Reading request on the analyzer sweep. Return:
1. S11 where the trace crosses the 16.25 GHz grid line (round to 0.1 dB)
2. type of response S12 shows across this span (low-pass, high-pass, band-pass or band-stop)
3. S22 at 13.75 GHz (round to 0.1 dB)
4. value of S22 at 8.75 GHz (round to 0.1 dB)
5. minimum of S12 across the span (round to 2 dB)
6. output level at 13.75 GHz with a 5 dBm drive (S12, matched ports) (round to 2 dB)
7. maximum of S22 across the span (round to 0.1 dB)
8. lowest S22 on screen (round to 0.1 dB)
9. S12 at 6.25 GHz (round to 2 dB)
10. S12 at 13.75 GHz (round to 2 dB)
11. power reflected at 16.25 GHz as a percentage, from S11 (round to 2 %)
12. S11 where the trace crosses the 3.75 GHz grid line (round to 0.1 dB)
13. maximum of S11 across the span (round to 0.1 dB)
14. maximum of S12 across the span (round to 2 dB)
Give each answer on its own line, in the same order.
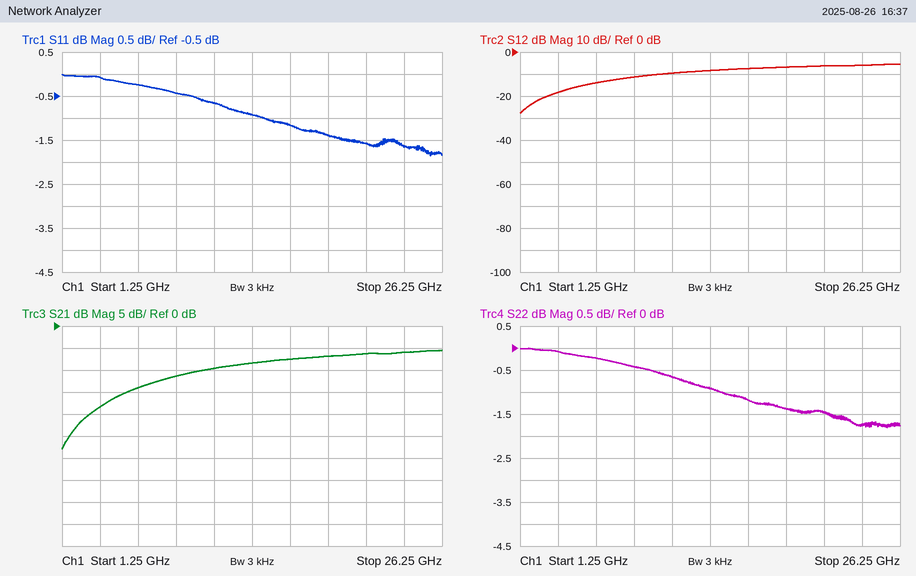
-1.2 dB
high-pass
-0.9 dB
-0.4 dB
-28 dB
-4 dBm
0.0 dB
-1.8 dB
-14 dB
-8 dB
76 %
-0.1 dB
0.0 dB
-6 dB
